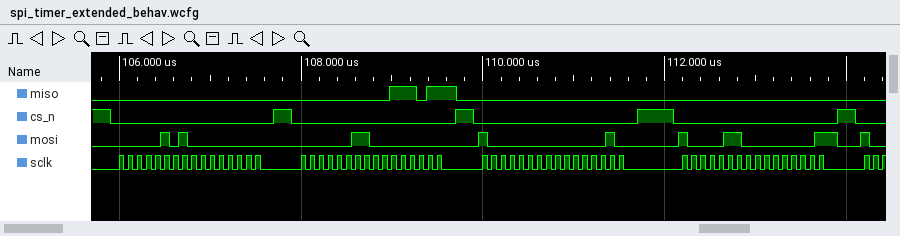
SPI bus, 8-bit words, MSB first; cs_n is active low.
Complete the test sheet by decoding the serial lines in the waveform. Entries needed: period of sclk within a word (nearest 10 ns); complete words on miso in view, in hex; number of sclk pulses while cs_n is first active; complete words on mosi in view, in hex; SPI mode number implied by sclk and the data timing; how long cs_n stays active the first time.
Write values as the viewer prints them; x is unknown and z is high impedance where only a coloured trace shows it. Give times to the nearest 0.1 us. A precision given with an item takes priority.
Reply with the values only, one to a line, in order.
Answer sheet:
100 ns
00, 00, 00, 3B, 00, 00, 00, 00
16
05, 00, 03, 00, 80, 02, 86, 01
0
1.8 us
